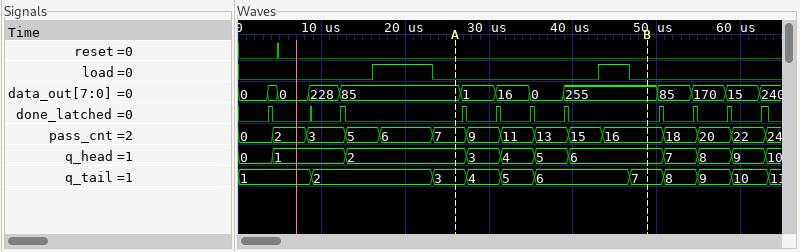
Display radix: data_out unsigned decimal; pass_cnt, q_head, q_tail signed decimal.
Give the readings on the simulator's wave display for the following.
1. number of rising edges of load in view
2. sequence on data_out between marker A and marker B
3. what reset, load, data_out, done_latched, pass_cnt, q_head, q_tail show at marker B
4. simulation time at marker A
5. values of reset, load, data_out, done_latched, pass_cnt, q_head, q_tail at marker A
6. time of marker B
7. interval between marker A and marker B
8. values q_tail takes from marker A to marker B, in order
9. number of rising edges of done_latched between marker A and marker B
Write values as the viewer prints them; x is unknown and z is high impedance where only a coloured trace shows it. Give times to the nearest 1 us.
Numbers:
2
85, 1, 16, 0, 255
reset=0, load=0, data_out=255, done_latched=0, pass_cnt=16, q_head=6, q_tail=7
26 us
reset=0, load=0, data_out=85, done_latched=0, pass_cnt=7, q_head=2, q_tail=3
49 us
23 us
3, 4, 5, 6, 7
4
